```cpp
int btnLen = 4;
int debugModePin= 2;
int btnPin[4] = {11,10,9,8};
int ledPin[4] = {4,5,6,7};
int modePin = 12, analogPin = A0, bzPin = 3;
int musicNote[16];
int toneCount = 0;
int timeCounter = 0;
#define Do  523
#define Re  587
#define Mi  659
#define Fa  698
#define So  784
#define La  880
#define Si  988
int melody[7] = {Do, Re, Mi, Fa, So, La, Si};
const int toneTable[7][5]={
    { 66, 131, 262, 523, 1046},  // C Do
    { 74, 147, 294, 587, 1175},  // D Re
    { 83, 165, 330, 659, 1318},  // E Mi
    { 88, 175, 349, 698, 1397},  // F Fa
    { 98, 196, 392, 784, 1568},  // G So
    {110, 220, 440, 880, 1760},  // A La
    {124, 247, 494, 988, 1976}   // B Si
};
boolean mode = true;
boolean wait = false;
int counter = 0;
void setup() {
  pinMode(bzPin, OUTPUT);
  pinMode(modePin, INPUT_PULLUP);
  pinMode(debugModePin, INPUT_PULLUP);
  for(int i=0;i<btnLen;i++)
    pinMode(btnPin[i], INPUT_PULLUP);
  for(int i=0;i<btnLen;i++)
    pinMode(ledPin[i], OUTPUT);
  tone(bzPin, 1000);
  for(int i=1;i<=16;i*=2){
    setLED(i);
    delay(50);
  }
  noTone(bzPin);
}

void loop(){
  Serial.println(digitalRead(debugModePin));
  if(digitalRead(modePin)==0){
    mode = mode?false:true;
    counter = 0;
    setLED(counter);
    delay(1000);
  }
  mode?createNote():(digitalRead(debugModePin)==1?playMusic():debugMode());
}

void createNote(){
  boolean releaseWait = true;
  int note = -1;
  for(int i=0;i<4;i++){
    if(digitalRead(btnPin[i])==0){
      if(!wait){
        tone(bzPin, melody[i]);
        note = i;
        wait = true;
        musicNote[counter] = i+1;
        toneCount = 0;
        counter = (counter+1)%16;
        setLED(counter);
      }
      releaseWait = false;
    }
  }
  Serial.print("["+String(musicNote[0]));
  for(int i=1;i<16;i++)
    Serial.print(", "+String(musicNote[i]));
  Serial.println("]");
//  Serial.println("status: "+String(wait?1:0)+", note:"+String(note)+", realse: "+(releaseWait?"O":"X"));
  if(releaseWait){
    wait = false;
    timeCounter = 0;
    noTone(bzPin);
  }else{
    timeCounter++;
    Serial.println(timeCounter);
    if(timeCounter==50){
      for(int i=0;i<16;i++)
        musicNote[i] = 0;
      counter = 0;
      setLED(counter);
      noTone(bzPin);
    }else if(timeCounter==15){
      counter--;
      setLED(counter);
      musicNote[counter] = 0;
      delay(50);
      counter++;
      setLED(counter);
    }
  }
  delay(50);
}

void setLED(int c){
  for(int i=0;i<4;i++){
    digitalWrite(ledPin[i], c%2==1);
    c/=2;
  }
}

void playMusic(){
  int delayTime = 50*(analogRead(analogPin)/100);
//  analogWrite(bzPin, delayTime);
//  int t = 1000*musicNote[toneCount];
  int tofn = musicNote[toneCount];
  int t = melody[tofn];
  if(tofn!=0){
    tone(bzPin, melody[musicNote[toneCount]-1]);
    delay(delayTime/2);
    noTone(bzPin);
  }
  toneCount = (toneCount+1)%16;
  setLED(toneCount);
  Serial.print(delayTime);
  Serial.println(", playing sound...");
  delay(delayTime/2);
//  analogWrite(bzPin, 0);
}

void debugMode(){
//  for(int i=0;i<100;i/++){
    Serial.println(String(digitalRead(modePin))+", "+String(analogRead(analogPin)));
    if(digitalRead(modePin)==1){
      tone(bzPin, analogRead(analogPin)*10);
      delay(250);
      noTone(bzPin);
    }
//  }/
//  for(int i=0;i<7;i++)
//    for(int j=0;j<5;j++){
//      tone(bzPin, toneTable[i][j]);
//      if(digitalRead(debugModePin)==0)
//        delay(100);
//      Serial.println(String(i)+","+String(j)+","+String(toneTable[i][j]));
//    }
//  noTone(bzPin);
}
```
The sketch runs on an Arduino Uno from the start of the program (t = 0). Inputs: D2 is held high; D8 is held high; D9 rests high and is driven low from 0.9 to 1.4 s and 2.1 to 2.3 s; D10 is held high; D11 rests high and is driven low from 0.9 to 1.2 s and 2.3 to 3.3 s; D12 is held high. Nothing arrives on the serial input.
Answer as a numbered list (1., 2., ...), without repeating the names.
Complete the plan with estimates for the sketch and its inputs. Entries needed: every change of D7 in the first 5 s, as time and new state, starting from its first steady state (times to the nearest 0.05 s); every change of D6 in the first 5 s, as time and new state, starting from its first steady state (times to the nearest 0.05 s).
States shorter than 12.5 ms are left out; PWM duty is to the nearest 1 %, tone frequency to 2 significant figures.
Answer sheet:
1. 0 s low; 0.15 s high; 0.2 s low
2. 0 s low; 0.1 s high; 0.15 s low
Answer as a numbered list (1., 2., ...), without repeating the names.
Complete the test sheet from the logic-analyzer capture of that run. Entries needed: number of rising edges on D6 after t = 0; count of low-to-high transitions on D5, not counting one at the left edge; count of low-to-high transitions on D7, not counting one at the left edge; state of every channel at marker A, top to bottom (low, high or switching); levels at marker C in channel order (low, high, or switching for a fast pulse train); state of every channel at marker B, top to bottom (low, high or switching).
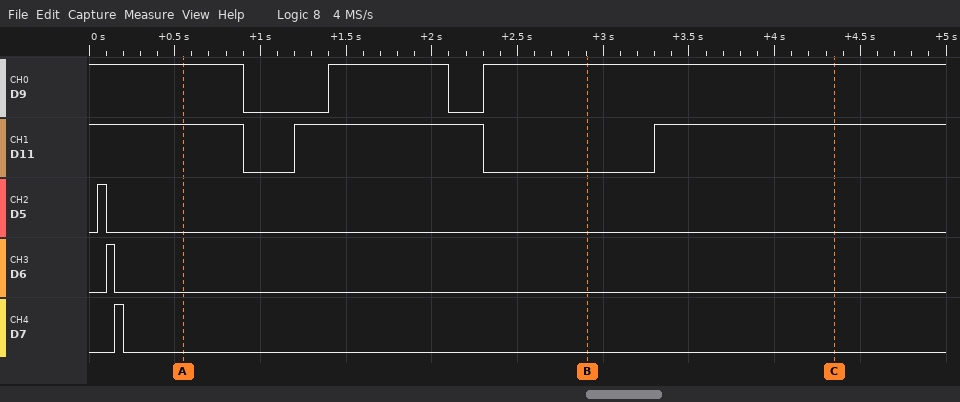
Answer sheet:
1. 1
2. 1
3. 1
4. D9 high, D11 high, D5 low, D6 low, D7 low
5. D9 high, D11 high, D5 low, D6 low, D7 low
6. D9 high, D11 low, D5 low, D6 low, D7 low
